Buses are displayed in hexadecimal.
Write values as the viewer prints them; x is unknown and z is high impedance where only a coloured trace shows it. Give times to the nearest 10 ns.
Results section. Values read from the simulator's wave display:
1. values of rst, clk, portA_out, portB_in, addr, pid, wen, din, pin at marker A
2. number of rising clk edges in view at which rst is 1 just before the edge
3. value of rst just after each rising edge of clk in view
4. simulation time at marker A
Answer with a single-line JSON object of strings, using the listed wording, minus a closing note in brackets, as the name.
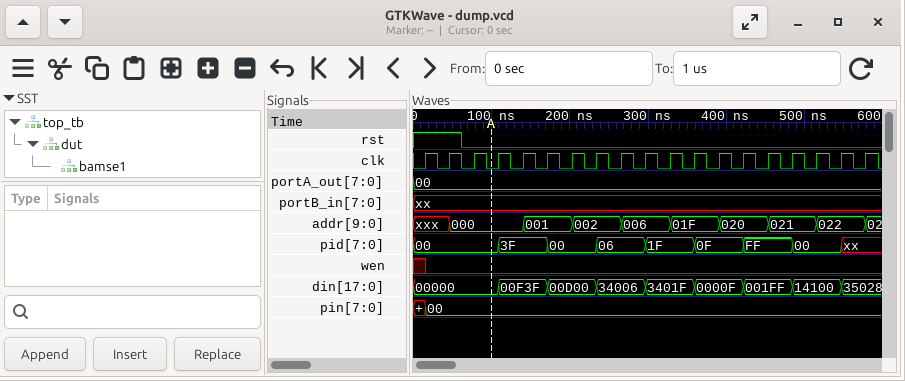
{"values of rst, clk, portA_out, portB_in, addr, pid, wen, din, pin at marker A": "rst=0, clk=0, portA_out=00, portB_in=xx, addr=000, pid=00, wen=0, din=00000, pin=00", "number of rising clk edges in view at which rst is 1 just before the edge": "2", "value of rst just after each rising edge of clk in view": "1 1 0 0 0 0 0 0 0 0 0 0 0 0 0 0 0 0 0", "simulation time at marker A": "100 ns"}
